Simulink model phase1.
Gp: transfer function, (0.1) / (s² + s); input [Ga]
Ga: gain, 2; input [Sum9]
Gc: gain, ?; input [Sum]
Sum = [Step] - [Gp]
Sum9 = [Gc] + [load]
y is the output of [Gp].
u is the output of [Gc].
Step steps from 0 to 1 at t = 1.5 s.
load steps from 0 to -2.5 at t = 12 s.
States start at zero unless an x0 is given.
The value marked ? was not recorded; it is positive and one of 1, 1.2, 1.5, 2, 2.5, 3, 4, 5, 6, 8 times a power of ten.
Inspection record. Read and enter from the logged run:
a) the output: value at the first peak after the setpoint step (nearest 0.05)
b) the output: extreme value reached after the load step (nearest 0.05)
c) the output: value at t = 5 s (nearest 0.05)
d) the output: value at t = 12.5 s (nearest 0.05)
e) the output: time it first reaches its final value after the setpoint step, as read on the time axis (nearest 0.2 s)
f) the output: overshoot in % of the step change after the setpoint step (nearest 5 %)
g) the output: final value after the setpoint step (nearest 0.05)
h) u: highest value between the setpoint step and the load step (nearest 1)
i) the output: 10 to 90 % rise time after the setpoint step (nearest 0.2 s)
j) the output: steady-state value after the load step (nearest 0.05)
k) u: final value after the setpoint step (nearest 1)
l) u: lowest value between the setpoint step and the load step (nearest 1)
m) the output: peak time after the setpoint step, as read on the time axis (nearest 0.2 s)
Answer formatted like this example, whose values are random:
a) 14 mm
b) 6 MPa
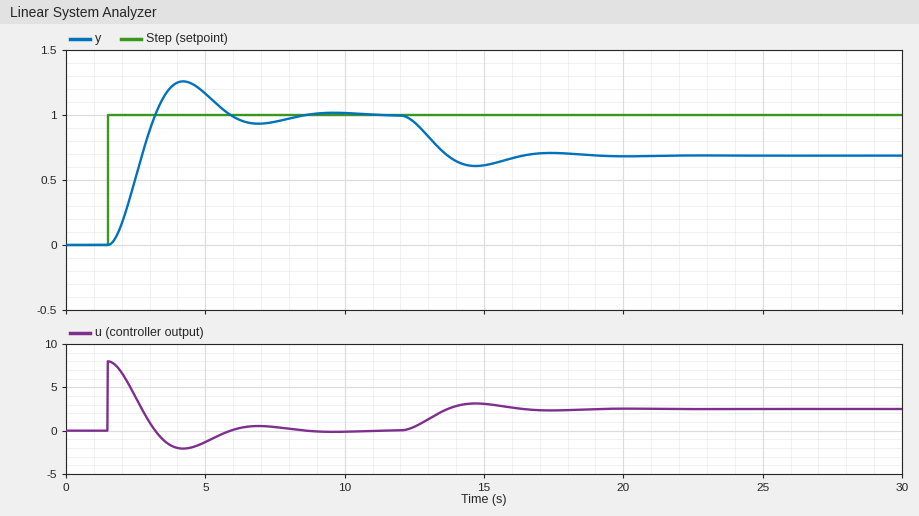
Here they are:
a) 1.25
b) 0.60
c) 1.15
d) 0.95
e) 3.2 s
f) 25 %
g) 1.00
h) 8
i) 1.2 s
j) 0.70
k) 0
l) -2
m) 4.2 s
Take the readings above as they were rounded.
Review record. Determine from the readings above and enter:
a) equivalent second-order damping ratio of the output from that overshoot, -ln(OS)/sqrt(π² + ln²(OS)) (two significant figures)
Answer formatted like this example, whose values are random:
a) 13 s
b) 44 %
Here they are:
a) 0.40
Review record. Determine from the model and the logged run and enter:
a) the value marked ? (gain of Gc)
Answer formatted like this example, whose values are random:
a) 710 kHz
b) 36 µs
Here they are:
a) 8
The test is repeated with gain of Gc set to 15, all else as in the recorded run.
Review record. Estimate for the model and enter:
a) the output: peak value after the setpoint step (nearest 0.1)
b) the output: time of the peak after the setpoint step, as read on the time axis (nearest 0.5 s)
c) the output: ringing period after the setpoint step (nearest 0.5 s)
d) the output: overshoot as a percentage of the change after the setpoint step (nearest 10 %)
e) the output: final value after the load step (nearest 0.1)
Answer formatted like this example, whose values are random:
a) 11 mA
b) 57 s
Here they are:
a) 1.4
b) 3.5 s
c) 4.0 s
d) 40 %
e) 0.8
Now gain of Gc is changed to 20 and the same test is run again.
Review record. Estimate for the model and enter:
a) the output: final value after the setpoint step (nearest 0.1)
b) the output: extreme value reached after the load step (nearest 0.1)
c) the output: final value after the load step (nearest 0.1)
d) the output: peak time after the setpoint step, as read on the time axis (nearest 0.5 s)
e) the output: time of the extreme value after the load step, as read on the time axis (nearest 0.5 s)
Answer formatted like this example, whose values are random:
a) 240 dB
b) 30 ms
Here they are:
a) 1.0
b) 0.8
c) 0.9
d) 3.0 s
e) 13.5 s
